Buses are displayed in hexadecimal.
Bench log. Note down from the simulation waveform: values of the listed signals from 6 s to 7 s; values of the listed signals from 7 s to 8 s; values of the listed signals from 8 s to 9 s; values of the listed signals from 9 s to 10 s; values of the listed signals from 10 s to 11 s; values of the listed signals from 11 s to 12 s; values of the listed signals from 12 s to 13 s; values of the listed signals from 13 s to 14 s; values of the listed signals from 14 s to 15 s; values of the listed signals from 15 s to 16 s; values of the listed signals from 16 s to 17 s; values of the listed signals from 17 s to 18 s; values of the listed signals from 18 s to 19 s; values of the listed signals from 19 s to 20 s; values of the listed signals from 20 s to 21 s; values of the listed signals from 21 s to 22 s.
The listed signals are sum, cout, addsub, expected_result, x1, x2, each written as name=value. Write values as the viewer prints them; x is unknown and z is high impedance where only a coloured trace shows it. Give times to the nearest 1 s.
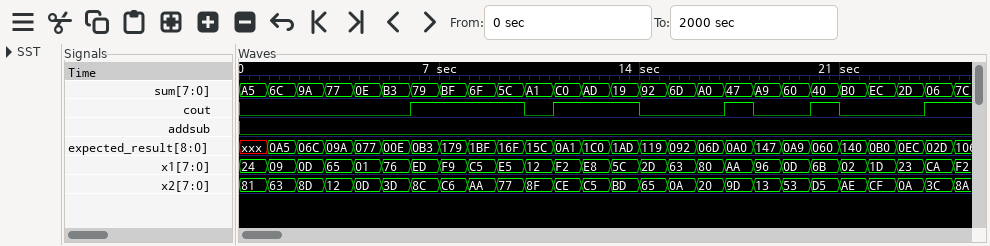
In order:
sum=79, cout=1, addsub=0, expected_result=0B3, x1=ED, x2=8C
sum=BF, cout=1, addsub=0, expected_result=179, x1=F9, x2=C6
sum=6F, cout=1, addsub=0, expected_result=1BF, x1=C5, x2=AA
sum=5C, cout=1, addsub=0, expected_result=16F, x1=E5, x2=77
sum=A1, cout=0, addsub=0, expected_result=15C, x1=12, x2=8F
sum=C0, cout=1, addsub=0, expected_result=0A1, x1=F2, x2=CE
sum=AD, cout=1, addsub=0, expected_result=1C0, x1=E8, x2=C5
sum=19, cout=1, addsub=0, expected_result=1AD, x1=5C, x2=BD
sum=92, cout=0, addsub=0, expected_result=119, x1=2D, x2=65
sum=6D, cout=0, addsub=0, expected_result=092, x1=63, x2=0A
sum=A0, cout=0, addsub=0, expected_result=06D, x1=80, x2=20
sum=47, cout=1, addsub=0, expected_result=0A0, x1=AA, x2=9D
sum=A9, cout=0, addsub=0, expected_result=147, x1=96, x2=13
sum=60, cout=0, addsub=0, expected_result=0A9, x1=0D, x2=53
sum=40, cout=1, addsub=0, expected_result=060, x1=6B, x2=D5
sum=B0, cout=0, addsub=0, expected_result=140, x1=02, x2=AE
